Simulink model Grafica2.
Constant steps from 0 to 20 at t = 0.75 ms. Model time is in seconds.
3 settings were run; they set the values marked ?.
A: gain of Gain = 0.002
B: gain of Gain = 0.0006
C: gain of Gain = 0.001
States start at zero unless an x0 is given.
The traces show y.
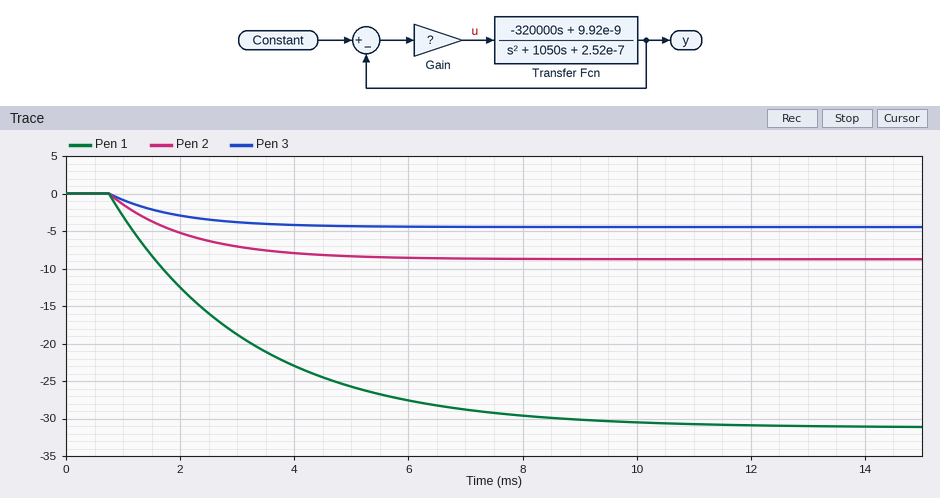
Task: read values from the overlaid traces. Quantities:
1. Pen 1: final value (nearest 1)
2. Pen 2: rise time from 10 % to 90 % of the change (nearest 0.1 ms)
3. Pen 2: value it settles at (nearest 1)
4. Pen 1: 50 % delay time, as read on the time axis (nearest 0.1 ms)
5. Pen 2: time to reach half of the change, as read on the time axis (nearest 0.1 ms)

-31
3.0 ms
-9
2.4 ms
1.7 ms
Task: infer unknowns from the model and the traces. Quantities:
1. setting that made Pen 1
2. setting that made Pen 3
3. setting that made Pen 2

A
B
C
